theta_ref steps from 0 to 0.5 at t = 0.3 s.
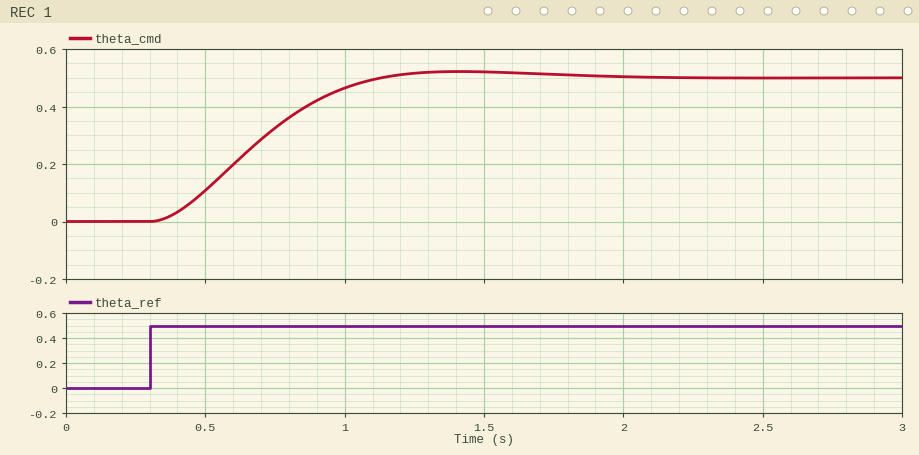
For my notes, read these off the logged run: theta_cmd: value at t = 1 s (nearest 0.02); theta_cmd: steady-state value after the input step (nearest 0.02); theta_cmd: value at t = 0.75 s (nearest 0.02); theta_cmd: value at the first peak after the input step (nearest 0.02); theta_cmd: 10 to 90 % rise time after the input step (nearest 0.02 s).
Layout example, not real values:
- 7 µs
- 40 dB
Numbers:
- 0.46
- 0.50
- 0.32
- 0.52
- 0.54 s
